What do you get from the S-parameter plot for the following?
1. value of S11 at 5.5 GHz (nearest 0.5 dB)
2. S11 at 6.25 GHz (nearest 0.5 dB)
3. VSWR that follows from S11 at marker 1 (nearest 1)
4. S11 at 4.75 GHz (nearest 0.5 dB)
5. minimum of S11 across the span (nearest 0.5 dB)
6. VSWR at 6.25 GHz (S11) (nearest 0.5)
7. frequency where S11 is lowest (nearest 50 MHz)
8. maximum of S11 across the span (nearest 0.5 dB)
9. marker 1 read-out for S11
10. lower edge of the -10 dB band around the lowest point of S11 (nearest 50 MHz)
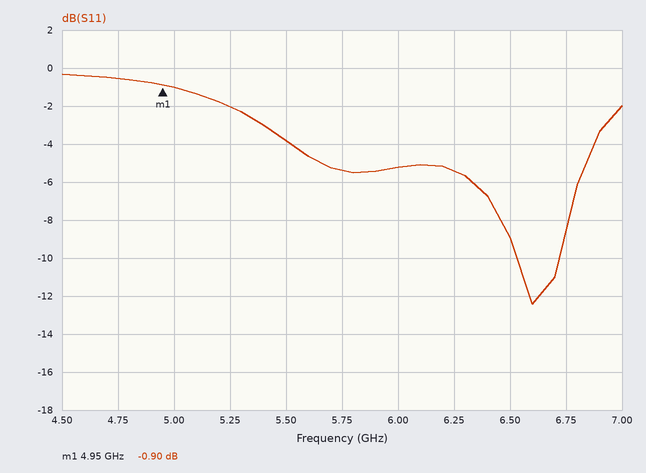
-4.0 dB
-5.5 dB
19
-0.5 dB
-12.5 dB
3.5
6.60 GHz
-0.5 dB
-0.90 dB
6.55 GHz
